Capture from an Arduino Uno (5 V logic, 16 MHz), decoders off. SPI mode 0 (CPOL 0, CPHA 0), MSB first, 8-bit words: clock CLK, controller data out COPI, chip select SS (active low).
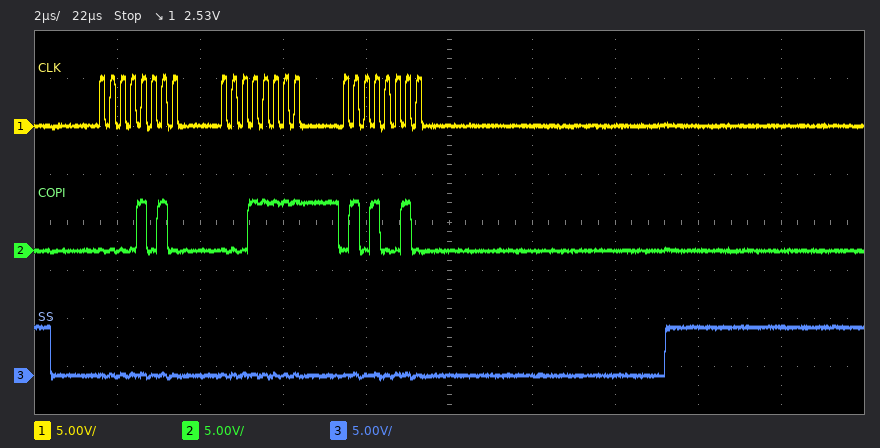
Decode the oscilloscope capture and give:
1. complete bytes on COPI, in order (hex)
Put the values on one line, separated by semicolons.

0A 1F 52
